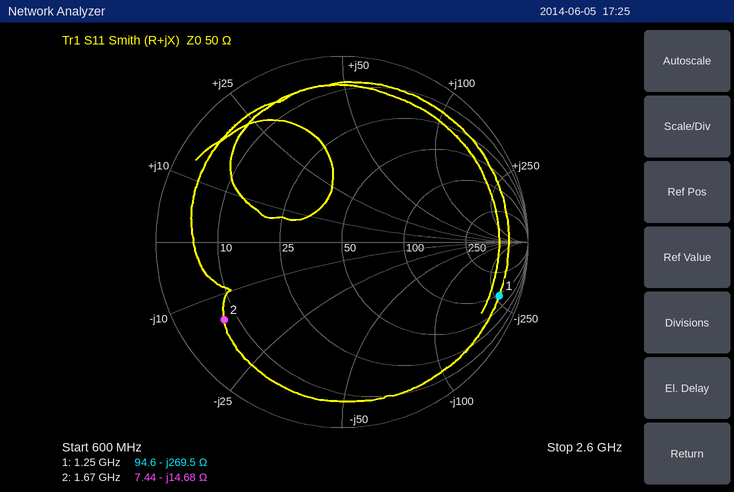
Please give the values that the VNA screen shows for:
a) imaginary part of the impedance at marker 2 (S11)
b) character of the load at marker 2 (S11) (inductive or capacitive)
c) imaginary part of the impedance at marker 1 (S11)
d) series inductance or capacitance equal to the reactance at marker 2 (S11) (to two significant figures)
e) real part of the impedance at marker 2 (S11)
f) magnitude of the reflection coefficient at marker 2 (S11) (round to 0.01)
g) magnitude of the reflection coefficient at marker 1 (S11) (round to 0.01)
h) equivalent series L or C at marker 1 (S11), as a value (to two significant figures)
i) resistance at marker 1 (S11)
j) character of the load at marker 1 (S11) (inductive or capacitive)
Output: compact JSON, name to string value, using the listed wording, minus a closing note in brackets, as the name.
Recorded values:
{"imaginary part of the impedance at marker 2": "-14.68 Ω", "character of the load at marker 2 (S11)": "capacitive", "imaginary part of the impedance at marker 1": "-269.5 Ω", "series inductance or capacitance equal to the reactance at marker 2 (S11)": "6.5 pF", "real part of the impedance at marker 2": "7.44 Ω", "magnitude of the reflection coefficient at marker 2 (S11)": "0.76", "magnitude of the reflection coefficient at marker 1 (S11)": "0.89", "equivalent series L or C at marker 1 (S11), as a value": "470 fF", "resistance at marker 1": "94.6 Ω", "character of the load at marker 1 (S11)": "capacitive"}
